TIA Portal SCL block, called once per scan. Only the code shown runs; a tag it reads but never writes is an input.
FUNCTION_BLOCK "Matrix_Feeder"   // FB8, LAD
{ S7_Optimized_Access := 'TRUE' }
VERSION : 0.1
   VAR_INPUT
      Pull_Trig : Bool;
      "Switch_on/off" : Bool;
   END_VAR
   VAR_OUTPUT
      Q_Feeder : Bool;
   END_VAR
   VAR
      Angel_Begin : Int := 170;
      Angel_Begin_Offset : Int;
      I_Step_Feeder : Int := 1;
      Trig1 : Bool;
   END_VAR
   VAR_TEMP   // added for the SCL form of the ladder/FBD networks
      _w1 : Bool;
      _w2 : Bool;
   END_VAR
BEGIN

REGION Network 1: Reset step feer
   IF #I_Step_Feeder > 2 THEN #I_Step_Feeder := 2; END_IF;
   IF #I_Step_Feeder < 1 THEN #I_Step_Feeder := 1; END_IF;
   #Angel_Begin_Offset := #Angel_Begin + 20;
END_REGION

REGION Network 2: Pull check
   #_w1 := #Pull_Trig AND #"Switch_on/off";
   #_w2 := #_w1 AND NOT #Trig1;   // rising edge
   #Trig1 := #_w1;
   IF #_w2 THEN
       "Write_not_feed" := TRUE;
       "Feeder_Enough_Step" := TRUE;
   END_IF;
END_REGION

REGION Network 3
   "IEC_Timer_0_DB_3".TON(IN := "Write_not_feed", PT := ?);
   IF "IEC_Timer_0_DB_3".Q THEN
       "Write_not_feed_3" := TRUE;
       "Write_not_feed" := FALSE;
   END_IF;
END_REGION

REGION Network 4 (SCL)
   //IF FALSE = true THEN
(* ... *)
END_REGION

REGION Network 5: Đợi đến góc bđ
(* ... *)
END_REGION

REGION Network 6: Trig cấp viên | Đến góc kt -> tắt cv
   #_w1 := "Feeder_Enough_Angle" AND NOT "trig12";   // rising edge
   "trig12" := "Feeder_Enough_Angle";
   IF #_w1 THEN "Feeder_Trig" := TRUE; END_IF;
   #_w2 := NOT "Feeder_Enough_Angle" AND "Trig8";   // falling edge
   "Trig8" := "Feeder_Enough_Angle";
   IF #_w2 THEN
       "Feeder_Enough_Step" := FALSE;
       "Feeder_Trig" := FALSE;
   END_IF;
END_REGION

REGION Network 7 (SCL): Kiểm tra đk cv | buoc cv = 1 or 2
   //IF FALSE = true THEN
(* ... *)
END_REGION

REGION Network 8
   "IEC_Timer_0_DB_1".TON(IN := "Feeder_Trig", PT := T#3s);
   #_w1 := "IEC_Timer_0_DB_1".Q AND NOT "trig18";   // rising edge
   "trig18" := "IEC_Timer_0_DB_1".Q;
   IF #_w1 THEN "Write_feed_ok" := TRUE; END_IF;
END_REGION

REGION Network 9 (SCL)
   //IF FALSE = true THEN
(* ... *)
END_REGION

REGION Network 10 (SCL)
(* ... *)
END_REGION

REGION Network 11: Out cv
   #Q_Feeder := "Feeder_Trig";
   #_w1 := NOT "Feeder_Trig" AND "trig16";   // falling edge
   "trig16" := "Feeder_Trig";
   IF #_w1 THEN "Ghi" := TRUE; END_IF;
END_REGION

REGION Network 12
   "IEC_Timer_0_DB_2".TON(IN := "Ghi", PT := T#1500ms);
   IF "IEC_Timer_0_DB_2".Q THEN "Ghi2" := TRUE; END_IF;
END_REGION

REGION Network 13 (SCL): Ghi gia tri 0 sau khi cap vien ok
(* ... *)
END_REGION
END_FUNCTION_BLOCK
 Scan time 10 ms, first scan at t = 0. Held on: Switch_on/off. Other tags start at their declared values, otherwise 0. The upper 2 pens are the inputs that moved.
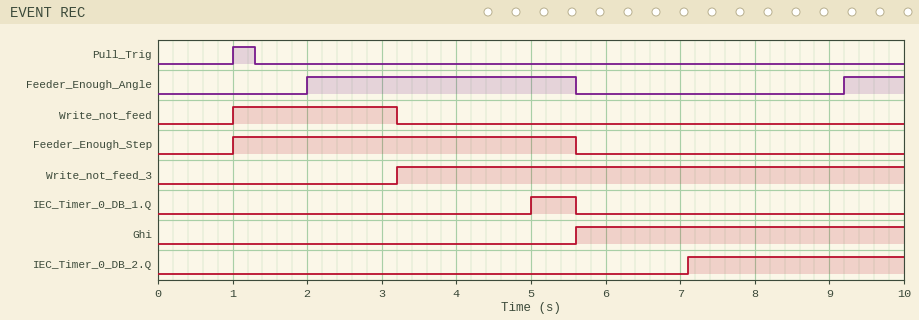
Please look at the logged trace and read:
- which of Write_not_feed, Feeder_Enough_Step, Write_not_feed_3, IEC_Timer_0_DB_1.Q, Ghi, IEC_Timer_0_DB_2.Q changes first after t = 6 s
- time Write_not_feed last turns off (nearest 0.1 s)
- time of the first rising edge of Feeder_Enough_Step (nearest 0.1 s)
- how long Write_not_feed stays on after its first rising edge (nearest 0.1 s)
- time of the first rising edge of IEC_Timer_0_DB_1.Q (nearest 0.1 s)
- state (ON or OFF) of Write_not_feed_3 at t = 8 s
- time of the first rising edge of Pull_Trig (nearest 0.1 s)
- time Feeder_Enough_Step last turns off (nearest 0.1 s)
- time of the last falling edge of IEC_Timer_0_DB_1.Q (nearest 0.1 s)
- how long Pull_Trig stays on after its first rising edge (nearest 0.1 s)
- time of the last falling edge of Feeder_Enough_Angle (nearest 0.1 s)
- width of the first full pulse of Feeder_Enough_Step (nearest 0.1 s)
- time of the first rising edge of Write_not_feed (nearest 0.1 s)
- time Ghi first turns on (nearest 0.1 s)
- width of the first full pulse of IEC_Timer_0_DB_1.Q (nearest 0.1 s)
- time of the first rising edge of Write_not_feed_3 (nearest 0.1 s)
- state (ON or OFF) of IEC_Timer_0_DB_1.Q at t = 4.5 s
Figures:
IEC_Timer_0_DB_2.Q
3.2 s
1.0 s
2.2 s
5.0 s
ON
1.0 s
5.6 s
5.6 s
0.3 s
5.6 s
4.6 s
1.0 s
5.6 s
0.6 s
3.2 s
OFF
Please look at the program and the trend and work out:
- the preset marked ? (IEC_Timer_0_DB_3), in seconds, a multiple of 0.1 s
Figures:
2.2 s
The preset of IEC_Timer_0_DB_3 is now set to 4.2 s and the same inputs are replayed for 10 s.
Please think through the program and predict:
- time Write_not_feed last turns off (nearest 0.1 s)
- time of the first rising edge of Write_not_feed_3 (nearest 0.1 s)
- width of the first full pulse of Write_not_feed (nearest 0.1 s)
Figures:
5.2 s
5.2 s
4.2 s
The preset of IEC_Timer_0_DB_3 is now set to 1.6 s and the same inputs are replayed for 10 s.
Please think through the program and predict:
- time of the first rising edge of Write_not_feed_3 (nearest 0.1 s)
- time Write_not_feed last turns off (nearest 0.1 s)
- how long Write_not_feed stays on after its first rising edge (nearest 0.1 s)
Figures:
2.6 s
2.6 s
1.6 s
